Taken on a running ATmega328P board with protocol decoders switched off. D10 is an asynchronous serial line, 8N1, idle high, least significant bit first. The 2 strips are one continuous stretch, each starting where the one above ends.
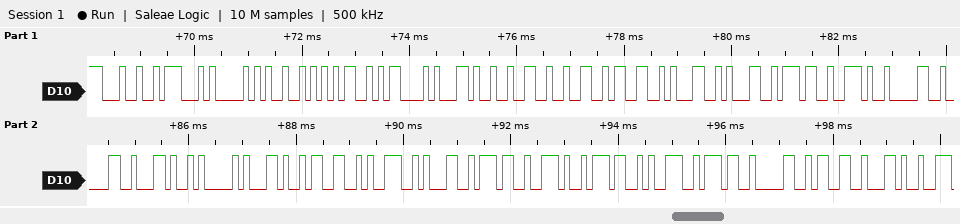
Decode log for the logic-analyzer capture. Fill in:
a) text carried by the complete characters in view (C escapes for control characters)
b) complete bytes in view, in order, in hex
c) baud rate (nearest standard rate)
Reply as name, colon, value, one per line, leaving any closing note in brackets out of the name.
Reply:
text carried by the complete characters in view: "$GPRMC,223117.00,A,3917.79703,"
complete bytes in view, in order, in hex: 0x24 0x47 0x50 0x52 0x4D 0x43 0x2C 0x32 0x32 0x33 0x31 0x31 0x37 0x2E 0x30 0x30 0x2C 0x41 0x2C 0x33 0x39 0x31 0x37 0x2E 0x37 0x39 0x37 0x30 0x33 0x2C
baud rate: 9600 baud
